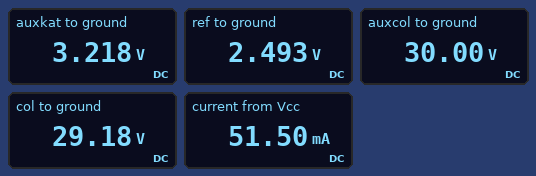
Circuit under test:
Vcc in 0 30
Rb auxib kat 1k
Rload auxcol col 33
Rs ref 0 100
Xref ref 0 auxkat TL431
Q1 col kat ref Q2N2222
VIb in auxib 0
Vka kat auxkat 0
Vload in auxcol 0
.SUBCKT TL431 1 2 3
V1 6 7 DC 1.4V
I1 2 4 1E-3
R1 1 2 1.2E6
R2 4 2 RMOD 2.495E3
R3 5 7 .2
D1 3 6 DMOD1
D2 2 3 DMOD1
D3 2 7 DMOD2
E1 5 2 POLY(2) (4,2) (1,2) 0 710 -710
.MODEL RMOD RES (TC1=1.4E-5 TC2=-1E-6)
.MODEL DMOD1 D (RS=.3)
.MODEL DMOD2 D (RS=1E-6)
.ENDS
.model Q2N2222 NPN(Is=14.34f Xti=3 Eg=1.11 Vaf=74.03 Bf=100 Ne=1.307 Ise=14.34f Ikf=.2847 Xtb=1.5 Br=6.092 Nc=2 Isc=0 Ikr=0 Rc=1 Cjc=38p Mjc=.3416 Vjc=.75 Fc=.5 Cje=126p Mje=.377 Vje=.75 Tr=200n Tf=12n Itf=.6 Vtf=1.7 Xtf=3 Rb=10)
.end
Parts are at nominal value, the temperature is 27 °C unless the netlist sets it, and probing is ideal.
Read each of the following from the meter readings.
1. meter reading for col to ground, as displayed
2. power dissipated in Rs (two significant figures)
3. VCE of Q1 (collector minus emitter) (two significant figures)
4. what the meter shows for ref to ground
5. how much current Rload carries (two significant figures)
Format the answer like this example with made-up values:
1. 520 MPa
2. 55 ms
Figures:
1. 29.18 V
2. 62 mW
3. 27 V
4. 2.493 V
5. 25 mA
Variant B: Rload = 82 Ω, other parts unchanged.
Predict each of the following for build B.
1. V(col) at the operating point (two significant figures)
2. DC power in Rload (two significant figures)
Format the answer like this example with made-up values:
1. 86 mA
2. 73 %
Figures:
1. 28 V
2. 50 mW
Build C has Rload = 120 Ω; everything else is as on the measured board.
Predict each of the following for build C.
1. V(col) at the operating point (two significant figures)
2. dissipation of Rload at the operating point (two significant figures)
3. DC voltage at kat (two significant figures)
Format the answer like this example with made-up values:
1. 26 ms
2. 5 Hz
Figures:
1. 27 V
2. 73 mW
3. 3.2 V
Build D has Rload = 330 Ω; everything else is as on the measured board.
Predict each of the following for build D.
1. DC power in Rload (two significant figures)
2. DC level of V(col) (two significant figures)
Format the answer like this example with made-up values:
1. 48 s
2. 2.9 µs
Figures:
1. 200 mW
2. 22 V
